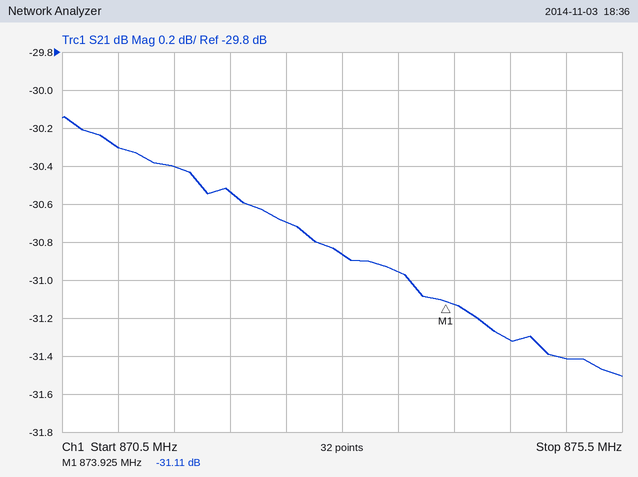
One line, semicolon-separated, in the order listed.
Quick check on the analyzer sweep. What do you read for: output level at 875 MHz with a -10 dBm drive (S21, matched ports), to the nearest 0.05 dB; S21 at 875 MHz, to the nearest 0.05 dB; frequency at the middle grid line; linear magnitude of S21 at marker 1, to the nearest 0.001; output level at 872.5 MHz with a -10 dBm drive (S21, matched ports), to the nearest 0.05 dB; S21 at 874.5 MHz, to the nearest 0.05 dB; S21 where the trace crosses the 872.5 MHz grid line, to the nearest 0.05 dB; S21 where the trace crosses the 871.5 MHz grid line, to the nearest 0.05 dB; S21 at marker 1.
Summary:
-41.40 dBm; -31.40 dB; 873 MHz; 0.028; -40.70 dBm; -31.30 dB; -30.70 dB; -30.40 dB; -31.11 dB
